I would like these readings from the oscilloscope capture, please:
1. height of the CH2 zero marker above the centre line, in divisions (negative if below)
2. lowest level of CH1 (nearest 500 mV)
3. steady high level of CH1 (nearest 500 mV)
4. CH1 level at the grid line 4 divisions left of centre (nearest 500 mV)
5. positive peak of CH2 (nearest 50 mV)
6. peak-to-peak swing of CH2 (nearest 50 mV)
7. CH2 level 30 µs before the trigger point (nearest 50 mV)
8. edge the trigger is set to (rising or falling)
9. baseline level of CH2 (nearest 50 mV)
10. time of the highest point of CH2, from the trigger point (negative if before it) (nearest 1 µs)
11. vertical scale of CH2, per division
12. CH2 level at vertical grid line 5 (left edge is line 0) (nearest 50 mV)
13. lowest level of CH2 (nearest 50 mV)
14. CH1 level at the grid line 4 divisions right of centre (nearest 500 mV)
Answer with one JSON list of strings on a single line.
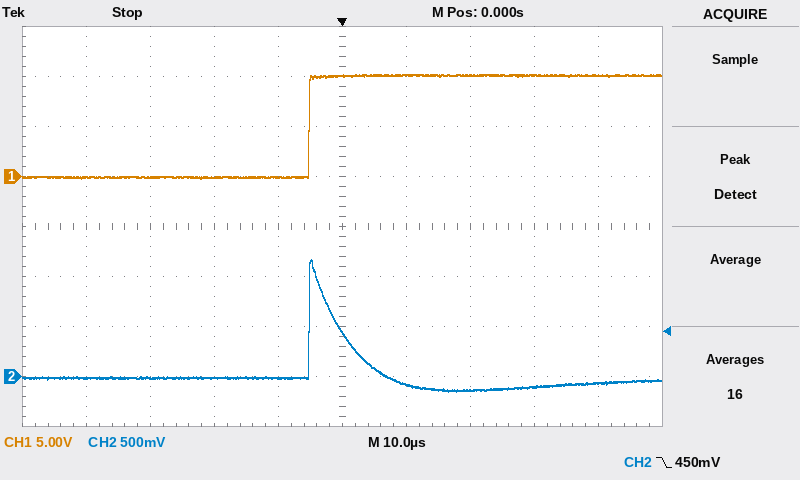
["-3.0 div", "0.0 V", "10.0 V", "0.0 V", "1.15 V", "1.30 V", "0 mV", "falling", "0 mV", "-5 µs", "500 mV", "450 mV", "-150 mV", "10.0 V"]
